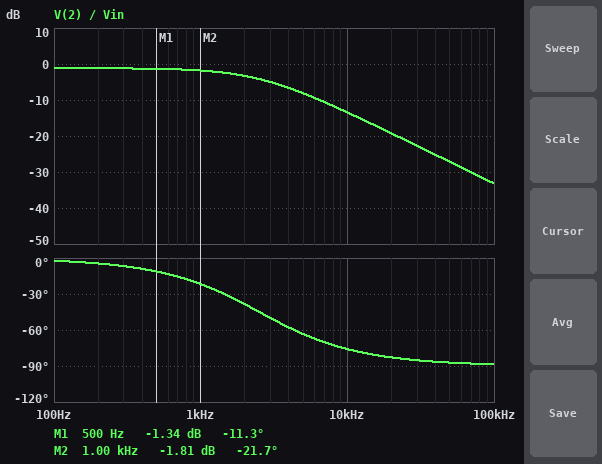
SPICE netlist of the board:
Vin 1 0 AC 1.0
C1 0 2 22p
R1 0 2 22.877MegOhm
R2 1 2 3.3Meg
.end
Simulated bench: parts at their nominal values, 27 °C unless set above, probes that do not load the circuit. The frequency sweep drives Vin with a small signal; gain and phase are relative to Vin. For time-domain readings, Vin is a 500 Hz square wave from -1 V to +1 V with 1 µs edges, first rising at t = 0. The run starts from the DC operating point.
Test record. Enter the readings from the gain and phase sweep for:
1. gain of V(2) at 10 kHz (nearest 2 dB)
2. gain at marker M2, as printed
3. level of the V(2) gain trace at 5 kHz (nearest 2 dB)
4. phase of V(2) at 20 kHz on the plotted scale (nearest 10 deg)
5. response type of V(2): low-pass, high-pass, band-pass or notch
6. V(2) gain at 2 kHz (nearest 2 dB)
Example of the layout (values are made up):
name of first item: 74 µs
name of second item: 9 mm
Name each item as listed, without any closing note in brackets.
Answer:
gain of V(2) at 10 kHz: -14 dB
gain at marker M2, as printed: -1.81 dB
level of the V(2) gain trace at 5 kHz: -8 dB
phase of V(2) at 20 kHz on the plotted scale: -80 deg
response type of V(2): low-pass, high-pass, band-pass or notch: low-pass
V(2) gain at 2 kHz: -4 dB
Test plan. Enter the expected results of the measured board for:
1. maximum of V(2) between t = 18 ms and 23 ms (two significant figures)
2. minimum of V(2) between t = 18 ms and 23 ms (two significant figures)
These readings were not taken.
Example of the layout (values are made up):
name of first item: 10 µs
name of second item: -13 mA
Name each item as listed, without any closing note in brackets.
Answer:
maximum of V(2) between t = 18 ms and 23 ms: 870 mV
minimum of V(2) between t = 18 ms and 23 ms: -870 mV
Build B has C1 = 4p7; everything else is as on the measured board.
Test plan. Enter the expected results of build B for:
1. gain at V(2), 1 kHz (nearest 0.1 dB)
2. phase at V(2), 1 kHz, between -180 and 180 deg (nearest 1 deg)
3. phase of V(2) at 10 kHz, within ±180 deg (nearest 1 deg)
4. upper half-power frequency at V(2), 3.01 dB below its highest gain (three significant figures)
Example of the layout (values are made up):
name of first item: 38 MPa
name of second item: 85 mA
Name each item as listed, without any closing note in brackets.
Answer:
gain at V(2), 1 kHz: -1.2 dB
phase at V(2), 1 kHz, between -180 and 180 deg: -5 deg
phase of V(2) at 10 kHz, within ±180 deg: -40 deg
upper half-power frequency at V(2), 3.01 dB below its highest gain: 11.7 kHz
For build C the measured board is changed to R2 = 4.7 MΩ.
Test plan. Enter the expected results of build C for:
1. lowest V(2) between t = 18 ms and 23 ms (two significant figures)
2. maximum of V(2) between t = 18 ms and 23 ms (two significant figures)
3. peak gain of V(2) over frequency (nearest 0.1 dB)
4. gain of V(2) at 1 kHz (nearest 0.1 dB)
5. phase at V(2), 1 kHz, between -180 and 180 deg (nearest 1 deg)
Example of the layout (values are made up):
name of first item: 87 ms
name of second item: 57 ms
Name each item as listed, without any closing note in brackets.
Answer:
lowest V(2) between t = 18 ms and 23 ms: -830 mV
maximum of V(2) between t = 18 ms and 23 ms: 830 mV
peak gain of V(2) over frequency: -1.6 dB
gain of V(2) at 1 kHz: -2.7 dB
phase at V(2), 1 kHz, between -180 and 180 deg: -28 deg
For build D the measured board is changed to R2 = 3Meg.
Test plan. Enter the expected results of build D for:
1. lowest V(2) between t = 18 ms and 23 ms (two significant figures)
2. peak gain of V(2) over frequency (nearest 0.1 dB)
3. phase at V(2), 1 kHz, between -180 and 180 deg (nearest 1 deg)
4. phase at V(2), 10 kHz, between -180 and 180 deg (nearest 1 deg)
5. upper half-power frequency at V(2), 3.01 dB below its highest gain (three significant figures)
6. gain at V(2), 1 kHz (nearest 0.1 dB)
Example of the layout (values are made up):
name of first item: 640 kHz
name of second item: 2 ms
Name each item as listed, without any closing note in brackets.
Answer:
lowest V(2) between t = 18 ms and 23 ms: -880 mV
peak gain of V(2) over frequency: -1.1 dB
phase at V(2), 1 kHz, between -180 and 180 deg: -20 deg
phase at V(2), 10 kHz, between -180 and 180 deg: -75 deg
upper half-power frequency at V(2), 3.01 dB below its highest gain: 2.73 kHz
gain at V(2), 1 kHz: -1.6 dB
